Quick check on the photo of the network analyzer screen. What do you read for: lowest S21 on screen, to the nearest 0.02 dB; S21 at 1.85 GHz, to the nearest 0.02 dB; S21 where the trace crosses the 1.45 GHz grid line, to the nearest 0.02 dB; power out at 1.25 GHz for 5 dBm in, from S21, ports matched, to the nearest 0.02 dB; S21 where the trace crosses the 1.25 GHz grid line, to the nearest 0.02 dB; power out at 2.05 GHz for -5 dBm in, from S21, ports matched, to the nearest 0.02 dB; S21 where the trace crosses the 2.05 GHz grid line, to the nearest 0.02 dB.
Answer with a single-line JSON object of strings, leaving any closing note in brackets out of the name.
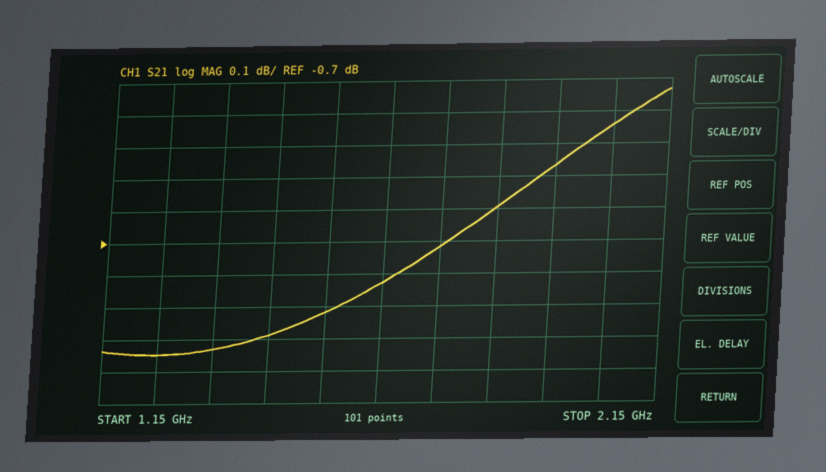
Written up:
{"lowest S21 on screen, to the nearest 0.02 dB": "-1.04 dB", "S21 at 1.85 GHz, to the nearest 0.02 dB": "-0.60 dB", "S21 where the trace crosses the 1.45 GHz grid line, to the nearest 0.02 dB": "-0.98 dB", "power out at 1.25 GHz for 5 dBm in, from S21, ports matched, to the nearest 0.02 dB": "3.96 dBm", "S21 where the trace crosses the 1.25 GHz grid line, to the nearest 0.02 dB": "-1.04 dB", "power out at 2.05 GHz for -5 dBm in, from S21, ports matched, to the nearest 0.02 dB": "-5.34 dBm", "S21 where the trace crosses the 2.05 GHz grid line, to the nearest 0.02 dB": "-0.34 dB"}
